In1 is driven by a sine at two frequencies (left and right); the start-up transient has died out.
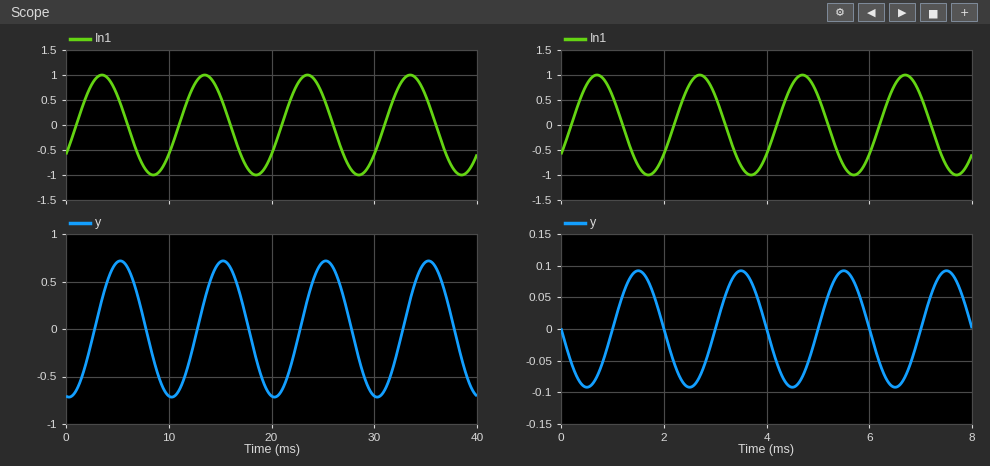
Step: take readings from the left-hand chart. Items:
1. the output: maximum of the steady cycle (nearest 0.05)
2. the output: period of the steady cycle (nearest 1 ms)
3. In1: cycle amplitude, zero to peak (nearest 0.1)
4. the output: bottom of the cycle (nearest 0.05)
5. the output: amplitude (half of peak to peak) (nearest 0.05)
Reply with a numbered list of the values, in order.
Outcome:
1. 0.70
2. 10 ms
3. 1.0
4. -0.70
5. 0.70
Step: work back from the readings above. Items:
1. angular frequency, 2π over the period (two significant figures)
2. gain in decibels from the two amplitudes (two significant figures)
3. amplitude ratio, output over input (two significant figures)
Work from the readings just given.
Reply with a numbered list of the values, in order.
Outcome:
1. 0.63 rad/ms
2. -3.1 dB
3. 0.70
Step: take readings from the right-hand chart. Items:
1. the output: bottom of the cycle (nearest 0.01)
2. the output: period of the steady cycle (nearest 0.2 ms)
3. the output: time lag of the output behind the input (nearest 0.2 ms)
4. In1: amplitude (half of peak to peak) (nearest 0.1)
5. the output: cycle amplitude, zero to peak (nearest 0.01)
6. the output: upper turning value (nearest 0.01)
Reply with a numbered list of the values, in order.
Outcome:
1. -0.09
2. 2.0 ms
3. 0.8 ms
4. 1.0
5. 0.09
6. 0.09
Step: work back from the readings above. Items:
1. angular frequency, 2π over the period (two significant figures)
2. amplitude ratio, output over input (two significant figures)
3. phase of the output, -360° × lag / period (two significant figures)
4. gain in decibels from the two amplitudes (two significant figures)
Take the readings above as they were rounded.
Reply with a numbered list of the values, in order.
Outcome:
1. 3.1 rad/ms
2. 0.090
3. -140°
4. -21 dB
